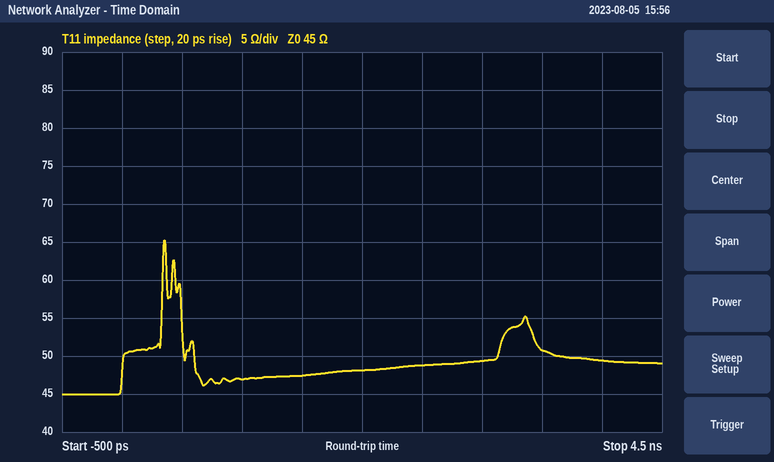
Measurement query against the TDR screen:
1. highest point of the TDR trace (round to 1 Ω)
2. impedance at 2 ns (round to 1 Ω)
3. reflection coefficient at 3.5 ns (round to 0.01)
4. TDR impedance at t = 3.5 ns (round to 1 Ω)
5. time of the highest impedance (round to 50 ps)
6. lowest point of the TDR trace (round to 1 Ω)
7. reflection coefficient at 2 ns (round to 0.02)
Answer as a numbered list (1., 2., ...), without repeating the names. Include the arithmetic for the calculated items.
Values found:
1. 65 Ω
2. 48 Ω
3. (51 − 45)/(51 + 45) ≈ +0.06
4. 51 Ω
5. 350 ps
6. 45 Ω
7. (48 − 45)/(48 + 45) ≈ +0.0323, so +0.04 to the nearest 0.02
